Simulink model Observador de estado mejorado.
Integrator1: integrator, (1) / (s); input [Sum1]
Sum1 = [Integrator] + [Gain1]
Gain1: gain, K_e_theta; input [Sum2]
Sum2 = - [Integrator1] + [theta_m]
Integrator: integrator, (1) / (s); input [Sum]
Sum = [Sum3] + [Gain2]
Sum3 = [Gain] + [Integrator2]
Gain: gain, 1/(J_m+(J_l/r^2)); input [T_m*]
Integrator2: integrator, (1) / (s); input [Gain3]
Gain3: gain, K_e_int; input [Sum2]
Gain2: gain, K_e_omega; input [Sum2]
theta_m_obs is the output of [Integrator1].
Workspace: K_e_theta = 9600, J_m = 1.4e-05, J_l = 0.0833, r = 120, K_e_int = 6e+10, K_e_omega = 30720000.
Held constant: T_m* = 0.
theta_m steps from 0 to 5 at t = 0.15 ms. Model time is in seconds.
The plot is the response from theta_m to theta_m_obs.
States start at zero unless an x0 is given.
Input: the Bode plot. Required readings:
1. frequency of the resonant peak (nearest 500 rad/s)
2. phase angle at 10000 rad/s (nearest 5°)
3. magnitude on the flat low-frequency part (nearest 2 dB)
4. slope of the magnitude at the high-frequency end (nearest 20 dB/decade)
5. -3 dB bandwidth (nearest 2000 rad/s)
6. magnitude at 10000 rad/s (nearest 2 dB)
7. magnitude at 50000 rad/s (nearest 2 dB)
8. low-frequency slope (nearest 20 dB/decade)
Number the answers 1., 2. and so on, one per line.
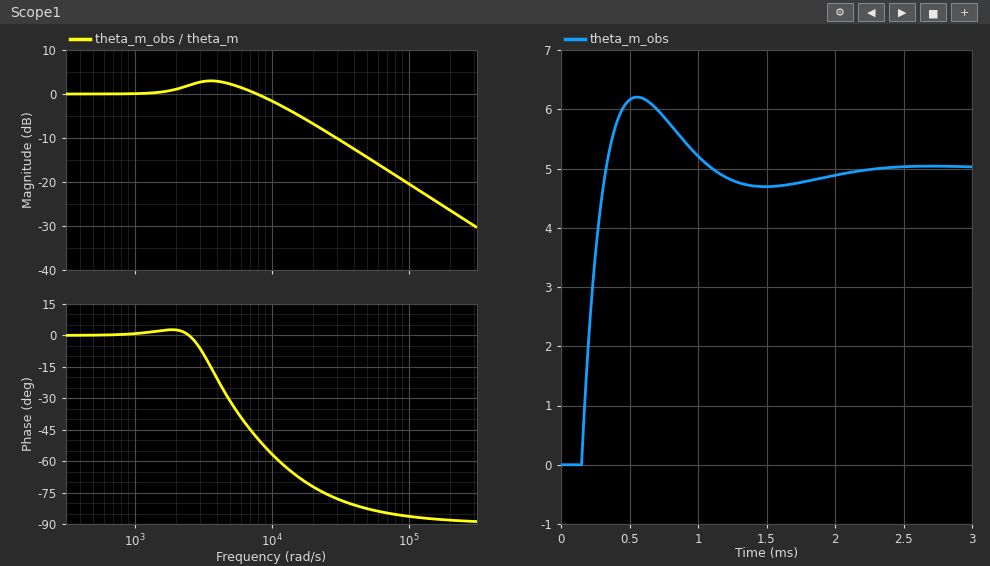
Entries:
1. 3500 rad/s
2. -55°
3. 0 dB
4. -20 dB/decade
5. 12000 rad/s
6. -2 dB
7. -14 dB
8. 0 dB/decade
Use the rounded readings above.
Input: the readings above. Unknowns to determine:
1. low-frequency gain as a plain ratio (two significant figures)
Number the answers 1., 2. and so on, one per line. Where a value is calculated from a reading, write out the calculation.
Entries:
1. 10^(0 / 20) = 1.0
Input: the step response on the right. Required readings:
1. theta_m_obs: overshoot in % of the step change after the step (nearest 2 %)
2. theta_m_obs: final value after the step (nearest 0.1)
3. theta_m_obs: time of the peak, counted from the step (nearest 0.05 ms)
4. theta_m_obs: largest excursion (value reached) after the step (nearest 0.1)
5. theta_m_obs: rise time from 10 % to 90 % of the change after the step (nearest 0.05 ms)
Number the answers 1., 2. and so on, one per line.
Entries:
1. 24 %
2. 5.0
3. 0.40 ms
4. 6.2
5. 0.15 ms
